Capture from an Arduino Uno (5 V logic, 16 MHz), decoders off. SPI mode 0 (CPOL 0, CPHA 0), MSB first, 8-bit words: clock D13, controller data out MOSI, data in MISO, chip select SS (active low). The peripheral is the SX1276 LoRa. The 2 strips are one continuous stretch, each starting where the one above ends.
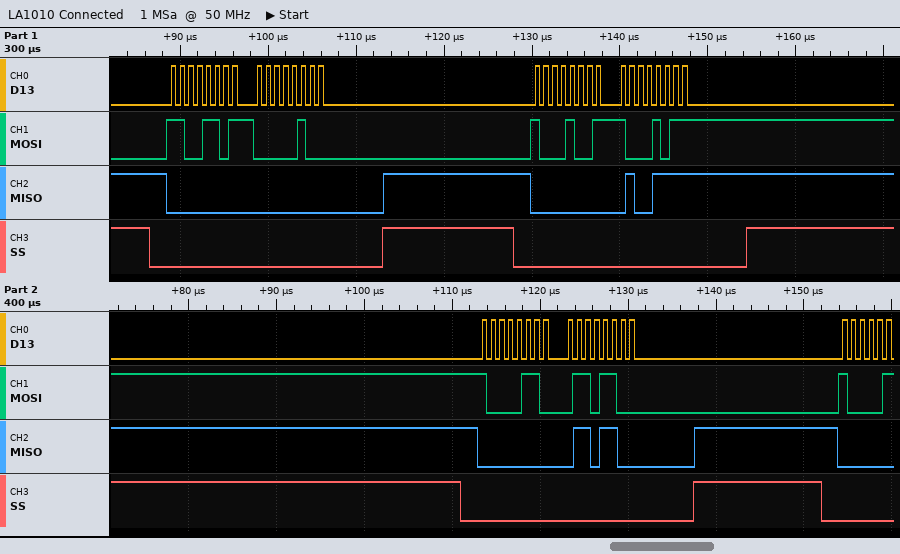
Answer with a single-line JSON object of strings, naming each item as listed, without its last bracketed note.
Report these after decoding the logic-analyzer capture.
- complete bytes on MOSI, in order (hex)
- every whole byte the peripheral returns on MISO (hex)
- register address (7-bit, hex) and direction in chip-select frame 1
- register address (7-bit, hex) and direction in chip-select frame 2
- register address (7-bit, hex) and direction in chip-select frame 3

{"complete bytes on MOSI, in order": "CD 04 89 8B 86 6C", "every whole byte the peripheral returns on MISO": "00 00 00 4F 00 6C", "register address (7-bit, hex) and direction in chip-select frame 1": "0x4D write", "register address (7-bit, hex) and direction in chip-select frame 2": "0x09 write", "register address (7-bit, hex) and direction in chip-select frame 3": "0x06 write"}
